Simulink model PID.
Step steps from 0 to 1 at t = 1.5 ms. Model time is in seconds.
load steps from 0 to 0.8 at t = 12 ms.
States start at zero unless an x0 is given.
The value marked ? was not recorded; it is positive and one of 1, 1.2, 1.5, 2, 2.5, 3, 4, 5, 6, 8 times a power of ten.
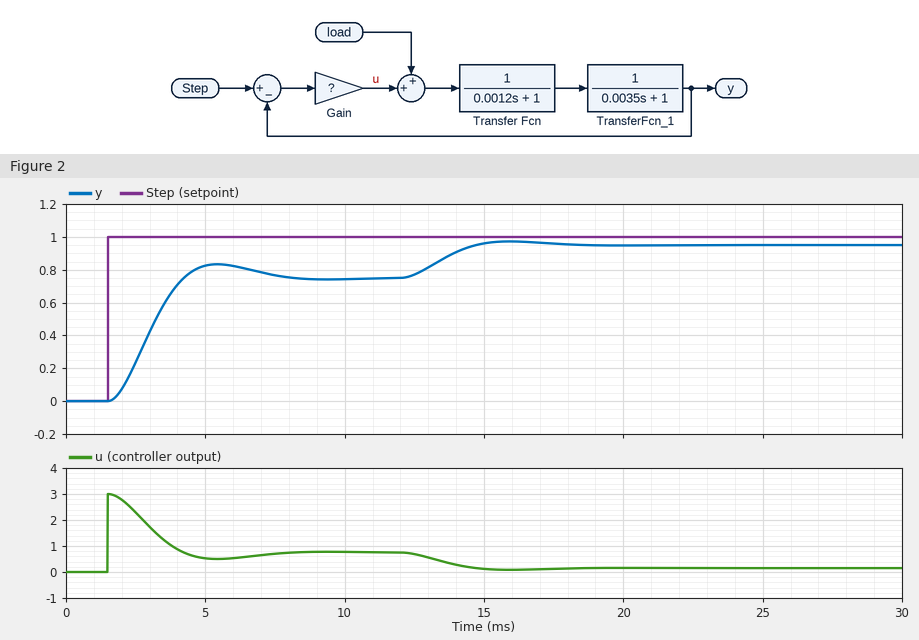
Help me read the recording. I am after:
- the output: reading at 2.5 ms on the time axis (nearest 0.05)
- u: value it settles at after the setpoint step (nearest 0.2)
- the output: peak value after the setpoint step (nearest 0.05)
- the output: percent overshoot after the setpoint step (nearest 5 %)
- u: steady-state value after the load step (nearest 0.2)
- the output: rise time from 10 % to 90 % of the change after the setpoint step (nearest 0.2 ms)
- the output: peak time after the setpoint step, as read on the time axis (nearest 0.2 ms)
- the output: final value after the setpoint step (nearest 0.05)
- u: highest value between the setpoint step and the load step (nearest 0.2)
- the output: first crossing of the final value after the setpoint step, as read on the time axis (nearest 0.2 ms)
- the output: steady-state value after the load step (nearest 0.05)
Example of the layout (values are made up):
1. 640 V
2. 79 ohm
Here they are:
1. 0.25
2. 0.8
3. 0.85
4. 10 %
5. 0.2
6. 1.8 ms
7. 5.4 ms
8. 0.75
9. 3.0
10. 4.2 ms
11. 0.95
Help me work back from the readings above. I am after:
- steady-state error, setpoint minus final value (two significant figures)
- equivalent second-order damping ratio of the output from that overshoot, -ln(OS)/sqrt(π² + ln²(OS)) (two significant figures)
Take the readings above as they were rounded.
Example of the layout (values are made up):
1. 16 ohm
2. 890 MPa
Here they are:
1. 0.25
2. 0.59
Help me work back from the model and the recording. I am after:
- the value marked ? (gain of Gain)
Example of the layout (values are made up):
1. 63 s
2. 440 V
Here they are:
1. 3
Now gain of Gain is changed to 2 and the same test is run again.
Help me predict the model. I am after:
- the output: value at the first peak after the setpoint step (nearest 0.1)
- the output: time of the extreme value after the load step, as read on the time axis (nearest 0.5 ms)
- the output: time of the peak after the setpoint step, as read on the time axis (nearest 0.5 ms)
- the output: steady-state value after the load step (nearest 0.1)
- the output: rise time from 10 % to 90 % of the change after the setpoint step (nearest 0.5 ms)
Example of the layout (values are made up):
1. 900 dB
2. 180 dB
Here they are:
1. 0.7
2. 17.0 ms
3. 6.5 ms
4. 0.9
5. 2.5 ms
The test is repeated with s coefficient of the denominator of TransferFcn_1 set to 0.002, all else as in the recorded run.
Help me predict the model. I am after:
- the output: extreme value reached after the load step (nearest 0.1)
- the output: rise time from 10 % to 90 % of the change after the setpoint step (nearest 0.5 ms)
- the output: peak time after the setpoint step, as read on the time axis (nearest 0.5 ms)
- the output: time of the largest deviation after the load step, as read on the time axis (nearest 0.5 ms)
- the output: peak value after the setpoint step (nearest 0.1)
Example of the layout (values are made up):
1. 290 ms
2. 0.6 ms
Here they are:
1. 1.0
2. 1.5 ms
3. 4.5 ms
4. 15.0 ms
5. 0.9
